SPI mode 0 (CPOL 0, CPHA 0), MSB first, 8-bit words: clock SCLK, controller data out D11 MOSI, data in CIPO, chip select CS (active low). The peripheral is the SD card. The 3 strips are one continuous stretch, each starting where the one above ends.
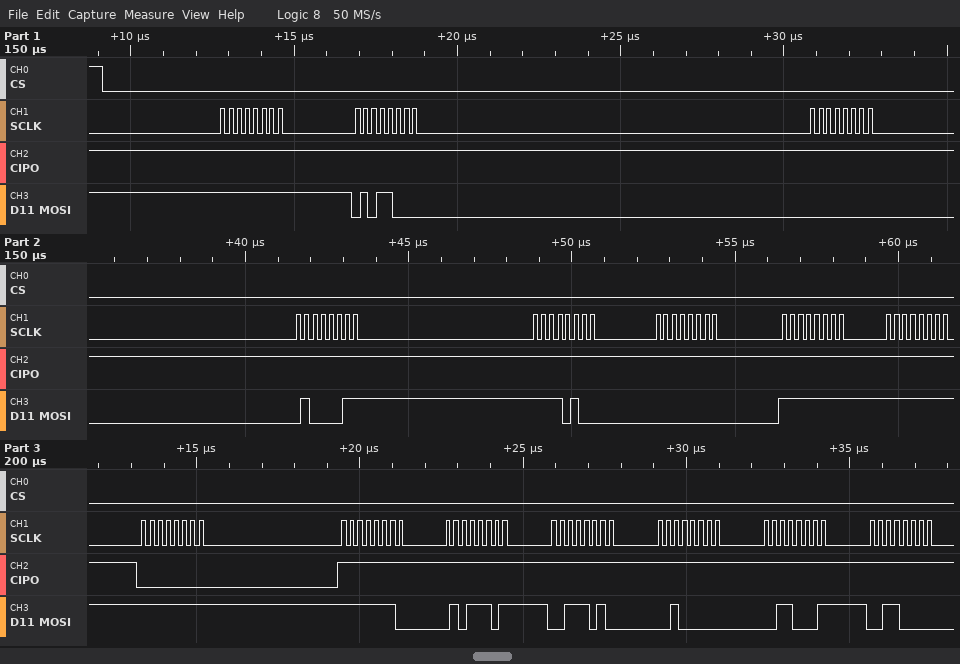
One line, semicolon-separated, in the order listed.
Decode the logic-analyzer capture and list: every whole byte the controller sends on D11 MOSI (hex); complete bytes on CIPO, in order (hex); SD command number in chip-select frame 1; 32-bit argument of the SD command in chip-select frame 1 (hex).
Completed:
FF 58 00 43 F4 00 FF FF FF FE 5D 3A 20 31 30; FF FF FF FF FF FF FF FF 00 FF FF FF FF FF FF; CMD24; 0x0043F400
